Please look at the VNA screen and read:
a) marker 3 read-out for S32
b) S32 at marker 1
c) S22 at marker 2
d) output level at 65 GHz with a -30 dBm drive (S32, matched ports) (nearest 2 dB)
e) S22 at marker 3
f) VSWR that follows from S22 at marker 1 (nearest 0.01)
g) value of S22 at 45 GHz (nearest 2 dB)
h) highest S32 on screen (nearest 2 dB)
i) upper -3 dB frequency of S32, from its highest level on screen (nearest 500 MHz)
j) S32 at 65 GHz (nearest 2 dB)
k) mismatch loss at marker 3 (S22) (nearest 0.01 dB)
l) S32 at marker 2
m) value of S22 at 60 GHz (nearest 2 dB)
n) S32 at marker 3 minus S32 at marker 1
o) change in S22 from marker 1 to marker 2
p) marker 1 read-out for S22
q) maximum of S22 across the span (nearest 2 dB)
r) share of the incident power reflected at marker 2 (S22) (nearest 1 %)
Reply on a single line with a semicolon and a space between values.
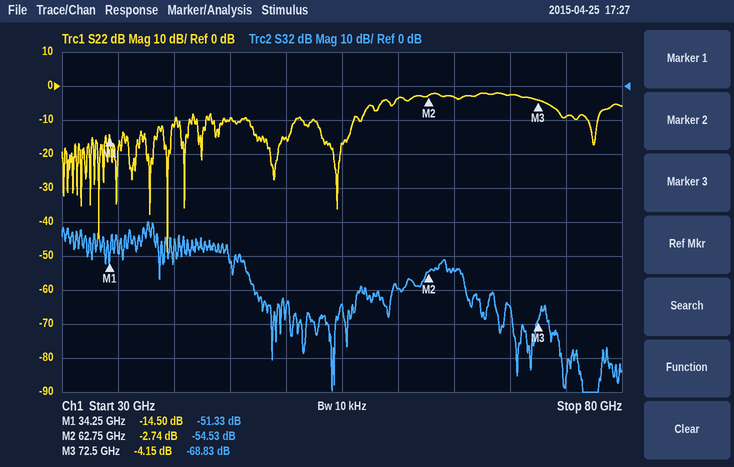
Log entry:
-68.83 dB; -51.33 dB; -2.74 dB; -84 dBm; -4.15 dB; 1.46; -10 dB; -40 dB; 38.0 GHz; -54 dB; 2.11 dB; -54.53 dB; -4 dB; -17.50 dB; 11.76 dB; -14.50 dB; -2 dB; 53 %
